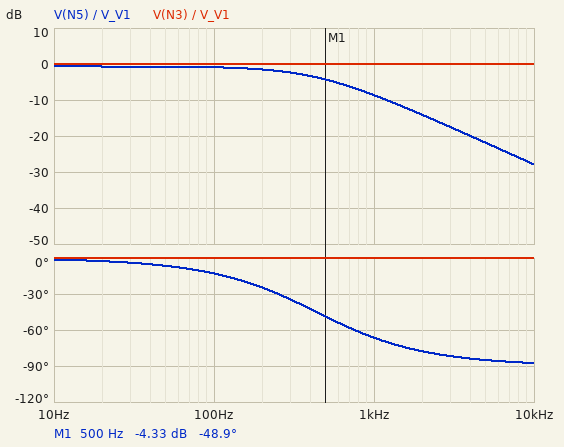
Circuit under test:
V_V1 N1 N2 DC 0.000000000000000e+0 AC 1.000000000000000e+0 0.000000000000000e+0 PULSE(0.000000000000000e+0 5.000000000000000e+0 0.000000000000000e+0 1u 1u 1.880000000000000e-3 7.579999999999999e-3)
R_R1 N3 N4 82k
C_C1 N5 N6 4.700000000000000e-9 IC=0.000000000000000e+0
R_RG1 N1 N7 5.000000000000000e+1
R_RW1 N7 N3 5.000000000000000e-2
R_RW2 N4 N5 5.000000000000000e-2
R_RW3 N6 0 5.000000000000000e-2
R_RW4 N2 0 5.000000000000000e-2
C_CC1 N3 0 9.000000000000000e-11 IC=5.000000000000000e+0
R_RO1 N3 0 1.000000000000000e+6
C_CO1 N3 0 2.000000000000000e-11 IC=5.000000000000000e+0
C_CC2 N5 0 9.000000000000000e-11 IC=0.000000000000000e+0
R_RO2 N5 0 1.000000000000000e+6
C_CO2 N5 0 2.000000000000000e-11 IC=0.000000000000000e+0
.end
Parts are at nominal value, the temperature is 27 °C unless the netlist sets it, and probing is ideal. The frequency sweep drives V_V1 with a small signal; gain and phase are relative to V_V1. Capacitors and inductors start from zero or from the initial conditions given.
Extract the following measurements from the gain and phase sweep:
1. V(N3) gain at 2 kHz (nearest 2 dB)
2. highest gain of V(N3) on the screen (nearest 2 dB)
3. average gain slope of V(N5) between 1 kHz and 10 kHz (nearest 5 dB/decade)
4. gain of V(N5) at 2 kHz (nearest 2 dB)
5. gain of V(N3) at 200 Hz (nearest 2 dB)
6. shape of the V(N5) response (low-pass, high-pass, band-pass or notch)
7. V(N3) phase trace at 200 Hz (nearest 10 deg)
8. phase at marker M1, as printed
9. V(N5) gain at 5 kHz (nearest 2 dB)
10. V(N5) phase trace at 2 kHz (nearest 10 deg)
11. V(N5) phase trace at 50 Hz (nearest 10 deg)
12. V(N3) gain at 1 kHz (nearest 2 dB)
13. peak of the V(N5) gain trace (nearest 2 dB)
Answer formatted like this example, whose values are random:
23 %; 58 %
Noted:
0 dB; 0 dB; -20 dB/decade; -14 dB; 0 dB; low-pass; 0 deg; -48.9 deg; -22 dB; -80 deg; -10 deg; 0 dB; 0 dB
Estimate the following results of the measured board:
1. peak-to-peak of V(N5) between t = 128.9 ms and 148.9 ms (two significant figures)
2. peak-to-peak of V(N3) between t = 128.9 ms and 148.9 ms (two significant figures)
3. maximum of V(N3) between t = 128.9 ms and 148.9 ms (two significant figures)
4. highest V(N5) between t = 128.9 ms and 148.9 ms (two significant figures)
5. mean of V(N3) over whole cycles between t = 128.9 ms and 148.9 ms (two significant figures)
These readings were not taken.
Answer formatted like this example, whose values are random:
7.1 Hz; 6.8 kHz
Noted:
4.6 V; 5.0 V; 5.0 V; 4.6 V; 1.2 V
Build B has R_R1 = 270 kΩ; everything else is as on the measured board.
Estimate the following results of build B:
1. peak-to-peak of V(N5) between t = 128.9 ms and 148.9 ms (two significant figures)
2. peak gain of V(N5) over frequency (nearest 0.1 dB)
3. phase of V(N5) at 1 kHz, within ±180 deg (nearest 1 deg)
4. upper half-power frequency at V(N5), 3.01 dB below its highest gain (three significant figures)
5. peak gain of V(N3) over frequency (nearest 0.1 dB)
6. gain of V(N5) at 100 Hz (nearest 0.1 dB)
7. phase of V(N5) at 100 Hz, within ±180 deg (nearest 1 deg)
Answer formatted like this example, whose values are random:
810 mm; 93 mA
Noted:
3.3 V; -2.1 dB; -81 deg; 156 Hz; 0 dB; -3.6 dB; -33 deg
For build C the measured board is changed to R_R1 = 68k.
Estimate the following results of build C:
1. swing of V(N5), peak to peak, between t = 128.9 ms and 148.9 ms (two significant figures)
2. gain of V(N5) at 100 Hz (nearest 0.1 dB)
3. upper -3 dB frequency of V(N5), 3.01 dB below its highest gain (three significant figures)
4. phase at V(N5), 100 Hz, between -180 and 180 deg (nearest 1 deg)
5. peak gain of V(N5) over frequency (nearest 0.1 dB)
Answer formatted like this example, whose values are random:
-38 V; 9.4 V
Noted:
4.7 V; -0.7 dB; 519 Hz; -11 deg; -0.6 dB
